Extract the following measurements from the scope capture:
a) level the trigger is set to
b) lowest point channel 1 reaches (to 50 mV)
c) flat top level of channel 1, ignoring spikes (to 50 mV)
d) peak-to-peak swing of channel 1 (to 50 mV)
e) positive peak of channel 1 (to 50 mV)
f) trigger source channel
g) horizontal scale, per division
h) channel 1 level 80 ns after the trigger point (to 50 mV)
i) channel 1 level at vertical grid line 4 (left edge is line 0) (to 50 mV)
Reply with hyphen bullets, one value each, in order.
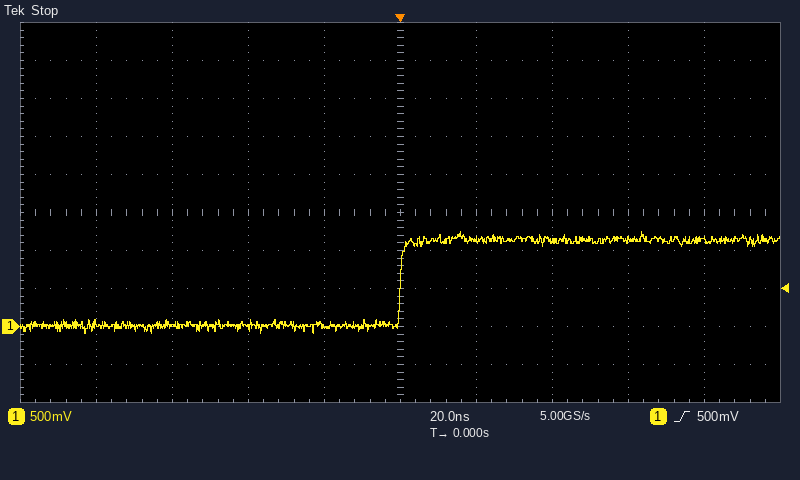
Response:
- 500 mV
- -100 mV
- 1.15 V
- 1.35 V
- 1.25 V
- channel 1
- 20 ns
- 1.15 V
- 0 mV
